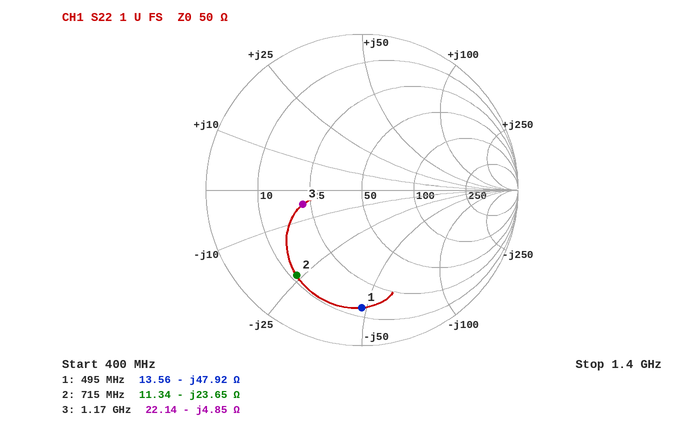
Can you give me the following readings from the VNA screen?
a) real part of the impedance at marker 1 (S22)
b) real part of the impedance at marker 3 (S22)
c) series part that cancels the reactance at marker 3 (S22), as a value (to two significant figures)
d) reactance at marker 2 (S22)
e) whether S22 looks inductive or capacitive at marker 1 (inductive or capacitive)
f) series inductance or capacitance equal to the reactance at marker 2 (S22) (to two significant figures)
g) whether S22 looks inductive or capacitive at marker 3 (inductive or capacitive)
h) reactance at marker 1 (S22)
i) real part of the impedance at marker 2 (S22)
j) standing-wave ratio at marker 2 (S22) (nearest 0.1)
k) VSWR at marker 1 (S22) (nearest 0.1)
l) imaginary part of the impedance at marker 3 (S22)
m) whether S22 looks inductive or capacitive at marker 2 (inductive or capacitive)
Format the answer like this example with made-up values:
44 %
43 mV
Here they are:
13.56 Ω
22.14 Ω
660 pH
-23.65 Ω
capacitive
9.4 pF
capacitive
-47.92 Ω
11.34 Ω
5.4
7.2
-4.85 Ω
capacitive
